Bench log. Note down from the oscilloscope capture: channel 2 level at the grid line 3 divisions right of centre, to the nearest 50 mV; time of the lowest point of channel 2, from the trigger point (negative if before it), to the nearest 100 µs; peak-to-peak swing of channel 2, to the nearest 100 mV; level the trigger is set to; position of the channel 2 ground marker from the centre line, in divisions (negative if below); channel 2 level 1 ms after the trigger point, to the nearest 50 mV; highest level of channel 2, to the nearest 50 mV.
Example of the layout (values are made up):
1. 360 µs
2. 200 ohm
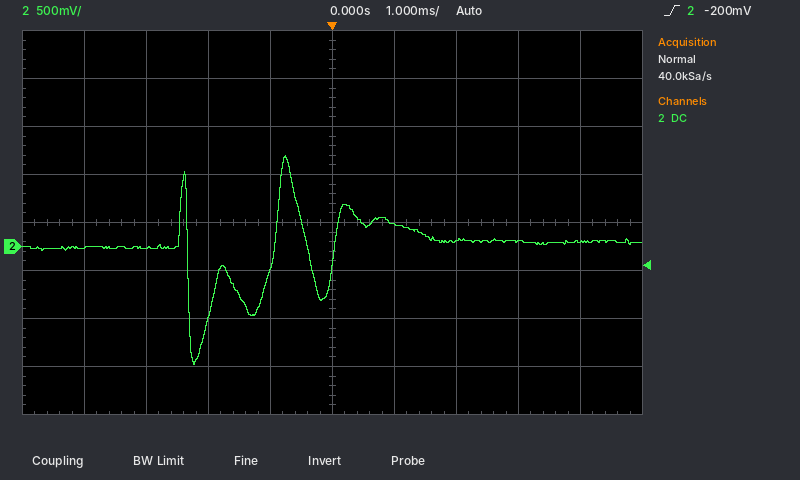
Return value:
1. 50 mV
2. -2.2 ms
3. 2.20 V
4. -200 mV
5. -0.5 div
6. 250 mV
7. 950 mV
